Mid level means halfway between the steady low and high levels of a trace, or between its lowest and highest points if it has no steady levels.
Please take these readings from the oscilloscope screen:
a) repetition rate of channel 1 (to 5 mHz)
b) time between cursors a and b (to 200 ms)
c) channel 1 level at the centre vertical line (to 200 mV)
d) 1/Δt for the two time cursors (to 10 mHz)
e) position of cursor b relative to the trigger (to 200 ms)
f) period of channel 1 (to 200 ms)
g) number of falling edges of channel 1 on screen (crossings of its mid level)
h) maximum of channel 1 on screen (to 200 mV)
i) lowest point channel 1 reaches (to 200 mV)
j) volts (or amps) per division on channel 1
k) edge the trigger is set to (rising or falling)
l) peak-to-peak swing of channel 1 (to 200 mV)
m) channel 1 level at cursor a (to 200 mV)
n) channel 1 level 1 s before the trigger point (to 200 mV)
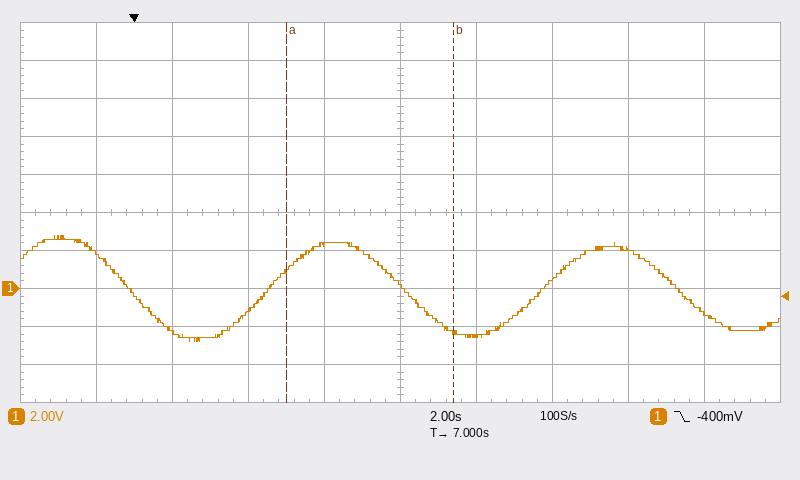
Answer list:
140 mHz
4.4 s
200 mV
230 mHz
+8.4 s
7.2 s
3
2.8 V
-2.8 V
2 V
falling
5.6 V
1.0 V
1.8 V
